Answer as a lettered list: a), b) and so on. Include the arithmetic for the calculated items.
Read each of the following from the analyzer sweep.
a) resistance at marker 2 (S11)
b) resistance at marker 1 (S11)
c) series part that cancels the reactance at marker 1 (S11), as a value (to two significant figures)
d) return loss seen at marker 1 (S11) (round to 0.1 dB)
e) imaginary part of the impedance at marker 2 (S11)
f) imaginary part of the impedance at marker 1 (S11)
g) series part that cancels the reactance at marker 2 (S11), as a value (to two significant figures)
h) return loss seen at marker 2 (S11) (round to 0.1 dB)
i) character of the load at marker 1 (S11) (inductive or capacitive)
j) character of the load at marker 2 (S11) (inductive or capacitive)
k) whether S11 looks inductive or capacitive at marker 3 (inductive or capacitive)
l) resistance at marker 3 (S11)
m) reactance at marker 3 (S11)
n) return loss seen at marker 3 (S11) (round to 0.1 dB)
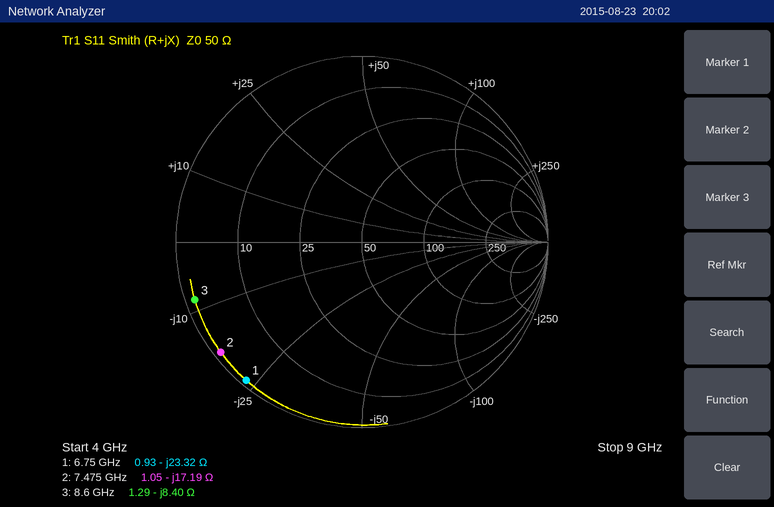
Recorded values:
a) 1.05 Ω
b) 0.93 Ω
c) L = 23.32 Ω/(2π × 6.75 GHz) ≈ 550 pH
d) 0.3 dB
e) -17.19 Ω
f) -23.32 Ω
g) L = 17.19 Ω/(2π × 7.475 GHz) ≈ 366 pH, so 370 pH to two significant figures
h) 0.3 dB
i) capacitive
j) capacitive
k) capacitive
l) 1.29 Ω
m) -8.40 Ω
n) 0.4 dB
